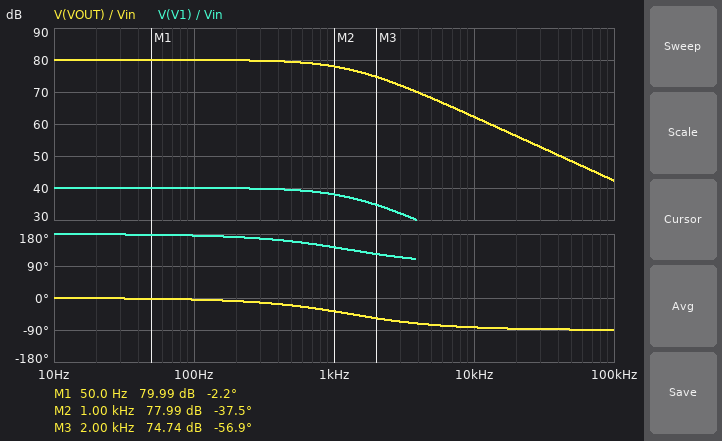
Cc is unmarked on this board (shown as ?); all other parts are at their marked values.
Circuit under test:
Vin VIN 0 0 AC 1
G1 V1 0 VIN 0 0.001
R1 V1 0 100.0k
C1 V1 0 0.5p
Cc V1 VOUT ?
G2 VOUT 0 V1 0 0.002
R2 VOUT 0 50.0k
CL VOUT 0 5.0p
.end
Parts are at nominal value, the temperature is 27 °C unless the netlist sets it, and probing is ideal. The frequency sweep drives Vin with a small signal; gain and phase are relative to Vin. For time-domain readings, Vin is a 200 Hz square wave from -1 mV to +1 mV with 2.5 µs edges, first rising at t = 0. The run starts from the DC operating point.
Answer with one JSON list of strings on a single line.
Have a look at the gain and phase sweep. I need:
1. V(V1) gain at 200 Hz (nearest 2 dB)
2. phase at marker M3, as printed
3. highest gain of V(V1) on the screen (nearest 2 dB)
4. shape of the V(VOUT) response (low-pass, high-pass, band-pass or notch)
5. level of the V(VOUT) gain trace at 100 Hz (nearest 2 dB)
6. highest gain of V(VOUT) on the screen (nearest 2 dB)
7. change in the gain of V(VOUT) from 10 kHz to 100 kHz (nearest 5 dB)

["40 dB", "-56.9 deg", "40 dB", "low-pass", "80 dB", "80 dB", "-20 dB"]
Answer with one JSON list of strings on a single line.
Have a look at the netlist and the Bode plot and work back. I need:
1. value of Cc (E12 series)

["12 pF"]
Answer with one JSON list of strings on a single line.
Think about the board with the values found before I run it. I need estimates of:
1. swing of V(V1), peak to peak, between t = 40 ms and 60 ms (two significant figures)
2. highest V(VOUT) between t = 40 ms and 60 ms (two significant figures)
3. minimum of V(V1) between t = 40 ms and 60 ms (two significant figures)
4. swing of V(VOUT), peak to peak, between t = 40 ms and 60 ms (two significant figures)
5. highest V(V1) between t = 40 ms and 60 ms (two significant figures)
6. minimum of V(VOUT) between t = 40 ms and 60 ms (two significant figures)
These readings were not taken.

["200 mV", "10 V", "-100 mV", "20 V", "100 mV", "-10 V"]
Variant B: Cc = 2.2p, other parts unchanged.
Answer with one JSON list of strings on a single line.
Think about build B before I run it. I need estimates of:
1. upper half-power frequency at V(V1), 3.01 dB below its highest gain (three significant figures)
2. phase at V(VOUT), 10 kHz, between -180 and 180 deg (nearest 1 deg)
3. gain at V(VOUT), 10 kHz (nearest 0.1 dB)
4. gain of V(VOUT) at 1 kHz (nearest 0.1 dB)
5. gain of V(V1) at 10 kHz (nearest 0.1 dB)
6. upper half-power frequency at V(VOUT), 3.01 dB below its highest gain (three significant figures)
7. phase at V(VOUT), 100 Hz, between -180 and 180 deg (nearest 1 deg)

["7.04 kHz", "-55 deg", "75.2 dB", "79.9 dB", "35.2 dB", "7.03 kHz", "-1 deg"]
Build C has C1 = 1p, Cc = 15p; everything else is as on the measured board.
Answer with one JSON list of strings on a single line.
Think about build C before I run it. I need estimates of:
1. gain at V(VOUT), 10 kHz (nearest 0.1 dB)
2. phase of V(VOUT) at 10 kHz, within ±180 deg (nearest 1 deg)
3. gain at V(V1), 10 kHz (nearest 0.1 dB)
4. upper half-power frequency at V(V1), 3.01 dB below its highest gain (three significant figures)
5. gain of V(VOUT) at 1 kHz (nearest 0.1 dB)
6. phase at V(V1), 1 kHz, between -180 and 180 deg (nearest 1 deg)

["60.3 dB", "-84 deg", "20.3 dB", "1.04 kHz", "77.2 dB", "137 deg"]
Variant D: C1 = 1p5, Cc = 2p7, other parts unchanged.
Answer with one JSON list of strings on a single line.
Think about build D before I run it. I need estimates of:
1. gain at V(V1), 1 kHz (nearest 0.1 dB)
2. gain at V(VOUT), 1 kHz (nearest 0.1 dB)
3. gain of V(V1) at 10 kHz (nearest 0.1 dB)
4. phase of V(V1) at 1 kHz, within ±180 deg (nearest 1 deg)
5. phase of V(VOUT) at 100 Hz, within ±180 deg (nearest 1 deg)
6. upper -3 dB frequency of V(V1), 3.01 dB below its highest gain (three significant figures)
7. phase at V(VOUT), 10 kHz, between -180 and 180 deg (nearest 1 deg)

["39.9 dB", "79.9 dB", "33.9 dB", "170 deg", "-1 deg", "5.73 kHz", "-60 deg"]
